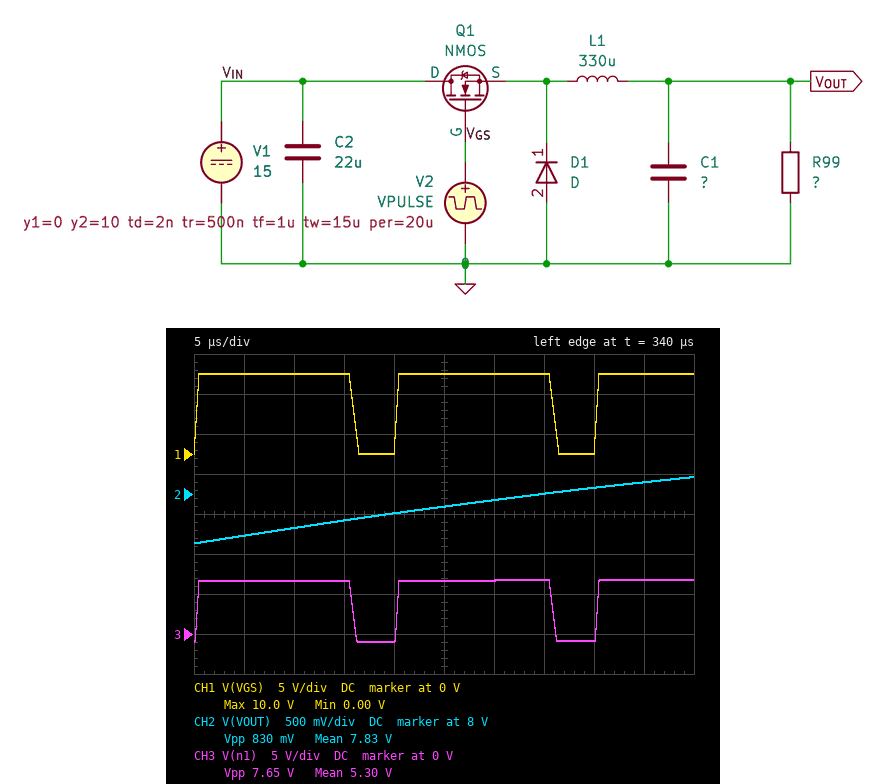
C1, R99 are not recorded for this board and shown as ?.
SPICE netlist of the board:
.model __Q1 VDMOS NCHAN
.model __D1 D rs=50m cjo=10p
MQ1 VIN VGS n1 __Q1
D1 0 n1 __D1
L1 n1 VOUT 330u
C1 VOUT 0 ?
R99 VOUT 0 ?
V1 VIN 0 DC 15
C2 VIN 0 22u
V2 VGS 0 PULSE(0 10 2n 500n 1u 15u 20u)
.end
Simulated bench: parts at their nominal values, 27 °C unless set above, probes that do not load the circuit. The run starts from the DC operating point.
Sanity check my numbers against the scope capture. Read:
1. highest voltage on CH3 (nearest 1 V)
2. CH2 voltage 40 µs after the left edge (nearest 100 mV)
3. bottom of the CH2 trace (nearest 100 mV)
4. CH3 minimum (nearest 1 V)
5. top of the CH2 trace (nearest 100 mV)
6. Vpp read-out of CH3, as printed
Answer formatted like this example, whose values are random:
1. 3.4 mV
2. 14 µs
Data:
1. 7 V
2. 8.1 V
3. 7.4 V
4. -1 V
5. 8.2 V
6. 7.65 V
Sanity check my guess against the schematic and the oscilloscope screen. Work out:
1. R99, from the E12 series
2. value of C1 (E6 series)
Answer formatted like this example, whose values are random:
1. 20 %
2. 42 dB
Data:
1. 12 Ω
2. 68 µF
